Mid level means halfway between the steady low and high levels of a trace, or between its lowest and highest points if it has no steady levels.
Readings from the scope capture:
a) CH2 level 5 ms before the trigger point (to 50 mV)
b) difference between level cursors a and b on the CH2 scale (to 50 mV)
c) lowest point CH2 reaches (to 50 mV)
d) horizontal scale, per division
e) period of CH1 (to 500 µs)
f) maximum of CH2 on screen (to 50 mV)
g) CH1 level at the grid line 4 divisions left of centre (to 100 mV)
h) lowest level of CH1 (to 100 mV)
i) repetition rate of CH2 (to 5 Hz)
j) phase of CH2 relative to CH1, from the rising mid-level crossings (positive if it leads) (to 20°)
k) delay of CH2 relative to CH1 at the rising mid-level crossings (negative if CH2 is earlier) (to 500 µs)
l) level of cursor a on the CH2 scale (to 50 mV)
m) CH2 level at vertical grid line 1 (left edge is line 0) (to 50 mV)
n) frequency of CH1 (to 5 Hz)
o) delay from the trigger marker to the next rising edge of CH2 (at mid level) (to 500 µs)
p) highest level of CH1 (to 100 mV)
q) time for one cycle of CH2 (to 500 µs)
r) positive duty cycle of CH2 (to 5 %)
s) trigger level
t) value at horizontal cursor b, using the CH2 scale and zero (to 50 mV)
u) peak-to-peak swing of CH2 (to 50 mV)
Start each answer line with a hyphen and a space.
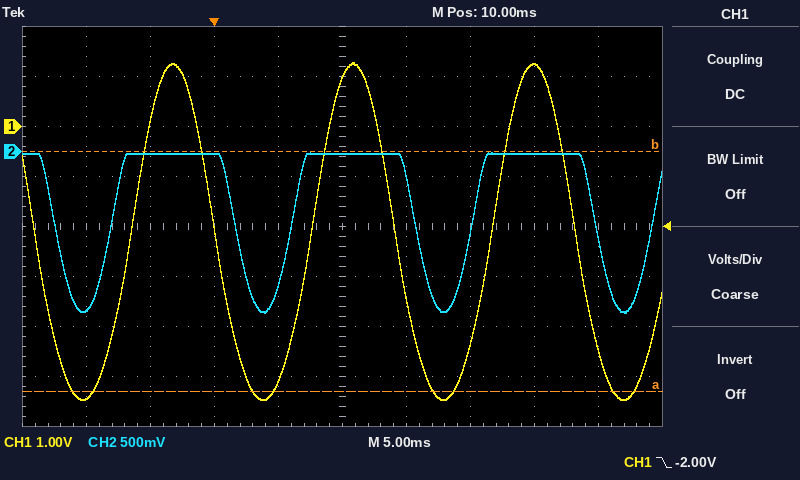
- 0 mV
- 2.40 V
- -1.60 V
- 5 ms
- 14.0 ms
- 0 mV
- -5.4 V
- -5.5 V
- 70 Hz
- +40°
- -1.5 ms
- -2.40 V
- -1.60 V
- 70 Hz
- 6.0 ms
- 1.3 V
- 14.0 ms
- 70 %
- -2.00 V
- 0 mV
- 1.60 V
